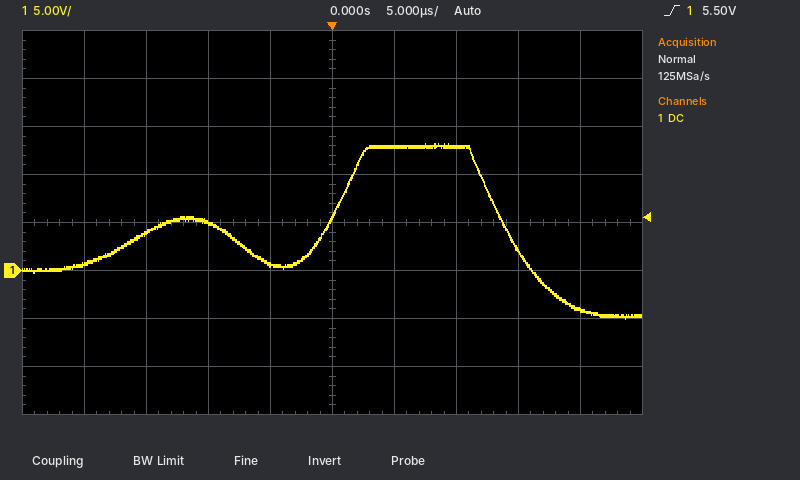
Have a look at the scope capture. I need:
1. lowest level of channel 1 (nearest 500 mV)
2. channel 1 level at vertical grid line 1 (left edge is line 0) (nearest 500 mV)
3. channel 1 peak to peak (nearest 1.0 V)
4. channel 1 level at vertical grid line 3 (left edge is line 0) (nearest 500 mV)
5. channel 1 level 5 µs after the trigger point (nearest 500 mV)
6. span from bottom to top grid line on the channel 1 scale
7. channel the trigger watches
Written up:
-5.0 V
500 mV
18.0 V
5.0 V
13.0 V
40 V
channel 1
